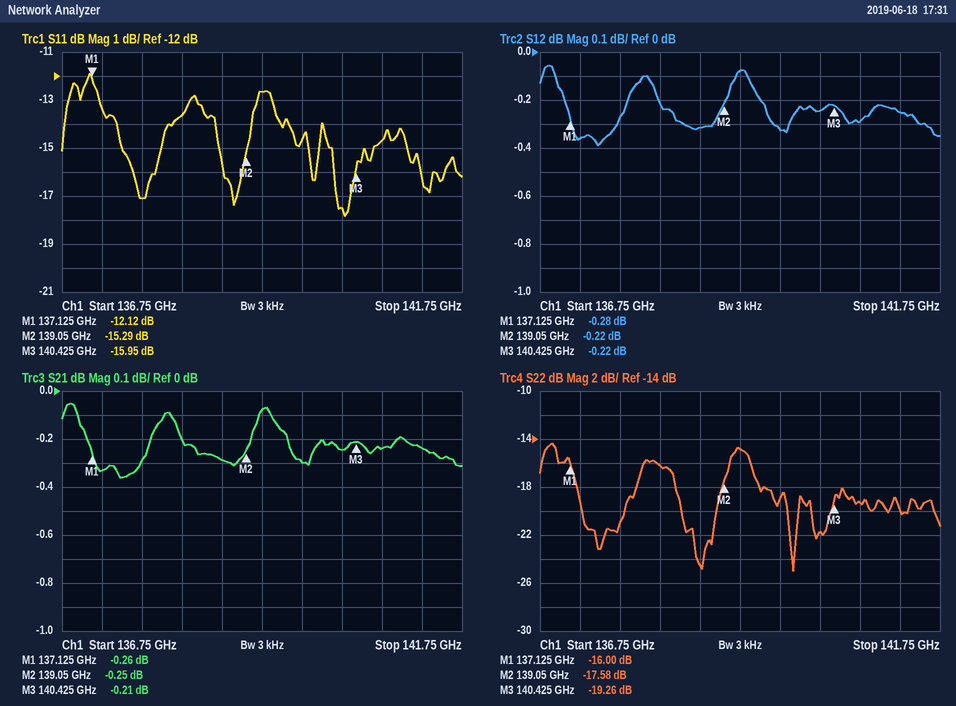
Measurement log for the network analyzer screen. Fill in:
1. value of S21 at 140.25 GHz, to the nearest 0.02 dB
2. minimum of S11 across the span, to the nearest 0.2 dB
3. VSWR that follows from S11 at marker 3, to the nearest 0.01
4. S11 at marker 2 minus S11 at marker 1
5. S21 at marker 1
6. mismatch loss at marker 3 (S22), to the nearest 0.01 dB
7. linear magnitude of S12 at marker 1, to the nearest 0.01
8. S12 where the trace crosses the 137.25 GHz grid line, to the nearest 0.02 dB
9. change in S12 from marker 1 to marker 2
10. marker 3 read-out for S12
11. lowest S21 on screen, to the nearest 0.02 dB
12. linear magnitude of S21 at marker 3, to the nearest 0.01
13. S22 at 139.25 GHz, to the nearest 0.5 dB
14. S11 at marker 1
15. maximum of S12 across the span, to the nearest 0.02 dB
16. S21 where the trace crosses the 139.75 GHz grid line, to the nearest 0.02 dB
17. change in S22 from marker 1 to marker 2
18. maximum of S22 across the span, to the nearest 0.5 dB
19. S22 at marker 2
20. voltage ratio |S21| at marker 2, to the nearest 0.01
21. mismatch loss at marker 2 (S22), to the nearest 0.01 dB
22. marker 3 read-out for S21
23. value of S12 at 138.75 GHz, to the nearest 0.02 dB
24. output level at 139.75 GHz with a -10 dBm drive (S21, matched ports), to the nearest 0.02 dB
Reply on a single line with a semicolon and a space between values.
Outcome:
-0.24 dB; -17.8 dB; 1.38; -3.17 dB; -0.26 dB; 0.05 dB; 0.97; -0.36 dB; 0.06 dB; -0.22 dB; -0.36 dB; 0.98; -15.0 dB; -12.12 dB; -0.06 dB; -0.30 dB; -1.58 dB; -14.5 dB; -17.58 dB; 0.97; 0.08 dB; -0.21 dB; -0.32 dB; -10.30 dBm
